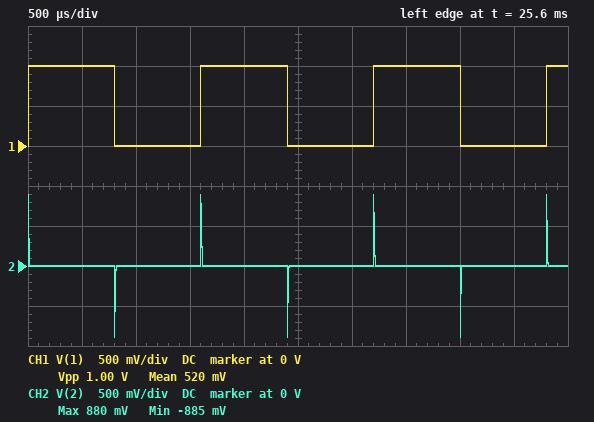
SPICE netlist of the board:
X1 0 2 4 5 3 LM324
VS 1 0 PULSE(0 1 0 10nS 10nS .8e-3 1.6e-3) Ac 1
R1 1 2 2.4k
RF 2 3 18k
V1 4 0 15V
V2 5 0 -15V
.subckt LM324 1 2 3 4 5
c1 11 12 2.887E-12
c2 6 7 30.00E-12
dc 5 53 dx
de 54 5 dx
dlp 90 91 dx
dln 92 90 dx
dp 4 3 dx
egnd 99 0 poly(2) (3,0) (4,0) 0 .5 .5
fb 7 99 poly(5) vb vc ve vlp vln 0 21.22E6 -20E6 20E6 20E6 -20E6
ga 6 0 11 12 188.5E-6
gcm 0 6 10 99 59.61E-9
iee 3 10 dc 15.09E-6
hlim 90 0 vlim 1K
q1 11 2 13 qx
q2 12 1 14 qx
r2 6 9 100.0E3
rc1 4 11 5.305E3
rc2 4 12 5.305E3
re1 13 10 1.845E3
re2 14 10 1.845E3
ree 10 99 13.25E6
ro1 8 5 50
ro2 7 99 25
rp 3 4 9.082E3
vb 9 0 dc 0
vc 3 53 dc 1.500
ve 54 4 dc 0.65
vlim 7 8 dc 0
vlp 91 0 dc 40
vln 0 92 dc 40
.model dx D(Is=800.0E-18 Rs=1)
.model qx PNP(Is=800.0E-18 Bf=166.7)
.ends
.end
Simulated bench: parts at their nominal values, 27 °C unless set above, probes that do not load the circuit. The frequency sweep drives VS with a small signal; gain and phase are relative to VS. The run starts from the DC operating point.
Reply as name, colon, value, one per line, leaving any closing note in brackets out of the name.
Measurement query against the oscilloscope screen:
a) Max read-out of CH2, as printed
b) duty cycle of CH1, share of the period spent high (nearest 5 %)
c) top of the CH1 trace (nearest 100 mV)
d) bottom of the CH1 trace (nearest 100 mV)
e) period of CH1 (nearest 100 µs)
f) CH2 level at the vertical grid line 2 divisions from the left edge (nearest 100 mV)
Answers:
Max read-out of CH2, as printed: 880 mV
duty cycle of CH1, share of the period spent high: 50 %
top of the CH1 trace: 1.0 V
bottom of the CH1 trace: 0 V
period of CH1: 1.6 ms
CH2 level at the vertical grid line 2 divisions from the left edge: 0 V
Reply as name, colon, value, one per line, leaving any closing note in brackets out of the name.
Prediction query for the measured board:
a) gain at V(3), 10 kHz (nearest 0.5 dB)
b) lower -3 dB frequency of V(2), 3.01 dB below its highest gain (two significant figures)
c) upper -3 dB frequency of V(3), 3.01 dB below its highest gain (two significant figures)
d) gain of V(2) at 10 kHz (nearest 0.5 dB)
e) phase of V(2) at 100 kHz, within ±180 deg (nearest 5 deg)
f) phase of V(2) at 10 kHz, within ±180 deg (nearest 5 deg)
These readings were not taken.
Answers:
gain at V(3), 10 kHz: 17.5 dB
lower -3 dB frequency of V(2), 3.01 dB below its highest gain: 120 kHz
upper -3 dB frequency of V(3), 3.01 dB below its highest gain: 120 kHz
gain of V(2) at 10 kHz: -22.5 dB
phase of V(2) at 100 kHz, within ±180 deg: 50 deg
phase of V(2) at 10 kHz, within ±180 deg: 85 deg
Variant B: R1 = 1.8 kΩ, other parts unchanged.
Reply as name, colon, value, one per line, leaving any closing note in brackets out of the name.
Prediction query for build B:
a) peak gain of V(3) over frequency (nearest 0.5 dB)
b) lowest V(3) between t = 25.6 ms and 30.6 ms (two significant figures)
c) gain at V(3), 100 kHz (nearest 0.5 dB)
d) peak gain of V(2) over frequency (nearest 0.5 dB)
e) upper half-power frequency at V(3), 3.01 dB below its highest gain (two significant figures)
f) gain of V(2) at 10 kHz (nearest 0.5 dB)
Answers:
peak gain of V(3) over frequency: 20.0 dB
lowest V(3) between t = 25.6 ms and 30.6 ms: -10 V
gain at V(3), 100 kHz: 16.5 dB
peak gain of V(2) over frequency: -0.5 dB
upper half-power frequency at V(3), 3.01 dB below its highest gain: 92 kHz
gain of V(2) at 10 kHz: -20.0 dB
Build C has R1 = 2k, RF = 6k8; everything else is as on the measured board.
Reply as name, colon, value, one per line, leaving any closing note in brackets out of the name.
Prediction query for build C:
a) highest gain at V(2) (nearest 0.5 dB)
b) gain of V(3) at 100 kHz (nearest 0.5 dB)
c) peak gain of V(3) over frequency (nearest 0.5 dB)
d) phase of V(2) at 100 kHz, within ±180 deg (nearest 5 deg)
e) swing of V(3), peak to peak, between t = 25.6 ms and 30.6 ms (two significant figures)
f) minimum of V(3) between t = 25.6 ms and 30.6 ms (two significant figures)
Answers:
highest gain at V(2): -2.0 dB
gain of V(3) at 100 kHz: 10.0 dB
peak gain of V(3) over frequency: 10.5 dB
phase of V(2) at 100 kHz, within ±180 deg: 65 deg
swing of V(3), peak to peak, between t = 25.6 ms and 30.6 ms: 3.4 V
minimum of V(3) between t = 25.6 ms and 30.6 ms: -3.4 V
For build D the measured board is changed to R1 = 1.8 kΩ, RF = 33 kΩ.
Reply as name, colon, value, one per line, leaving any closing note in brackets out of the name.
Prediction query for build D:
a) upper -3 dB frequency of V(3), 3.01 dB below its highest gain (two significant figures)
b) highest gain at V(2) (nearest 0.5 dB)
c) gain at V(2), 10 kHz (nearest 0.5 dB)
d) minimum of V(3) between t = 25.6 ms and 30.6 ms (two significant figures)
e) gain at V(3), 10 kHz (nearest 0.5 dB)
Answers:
upper -3 dB frequency of V(3), 3.01 dB below its highest gain: 52 kHz
highest gain at V(2): -0.5 dB
gain at V(2), 10 kHz: -15.0 dB
minimum of V(3) between t = 25.6 ms and 30.6 ms: -15 V
gain at V(3), 10 kHz: 25.0 dB
